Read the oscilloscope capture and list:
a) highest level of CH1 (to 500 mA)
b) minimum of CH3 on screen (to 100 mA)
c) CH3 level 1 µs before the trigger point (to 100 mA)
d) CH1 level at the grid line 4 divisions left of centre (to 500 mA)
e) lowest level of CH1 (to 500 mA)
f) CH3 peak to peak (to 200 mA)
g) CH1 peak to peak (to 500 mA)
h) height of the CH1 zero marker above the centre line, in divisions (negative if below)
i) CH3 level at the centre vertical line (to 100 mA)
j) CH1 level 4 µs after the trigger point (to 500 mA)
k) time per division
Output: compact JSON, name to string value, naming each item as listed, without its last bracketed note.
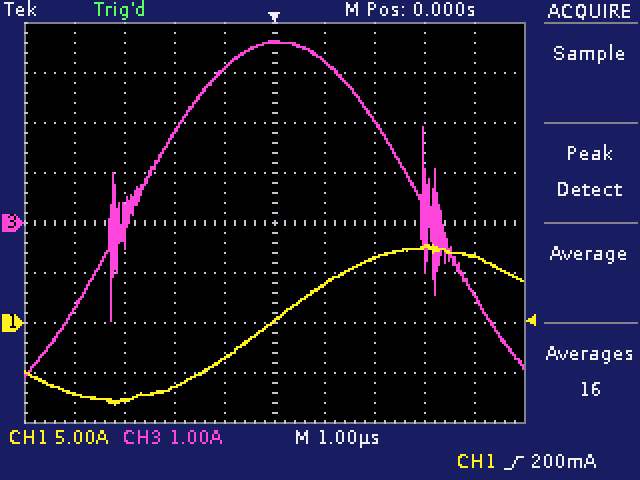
{"highest level of CH1": "8.0 A", "minimum of CH3 on screen": "-3.1 A", "CH3 level 1 µs before the trigger point": "3.1 A", "CH1 level at the grid line 4 divisions left of centre": "-7.0 A", "lowest level of CH1": "-8.0 A", "CH3 peak to peak": "6.8 A", "CH1 peak to peak": "16.0 A", "height of the CH1 zero marker above the centre line, in divisions": "-2.0 div", "CH3 level at the centre vertical line": "3.6 A", "CH1 level 4 µs after the trigger point": "6.5 A", "time per division": "1 µs"}
